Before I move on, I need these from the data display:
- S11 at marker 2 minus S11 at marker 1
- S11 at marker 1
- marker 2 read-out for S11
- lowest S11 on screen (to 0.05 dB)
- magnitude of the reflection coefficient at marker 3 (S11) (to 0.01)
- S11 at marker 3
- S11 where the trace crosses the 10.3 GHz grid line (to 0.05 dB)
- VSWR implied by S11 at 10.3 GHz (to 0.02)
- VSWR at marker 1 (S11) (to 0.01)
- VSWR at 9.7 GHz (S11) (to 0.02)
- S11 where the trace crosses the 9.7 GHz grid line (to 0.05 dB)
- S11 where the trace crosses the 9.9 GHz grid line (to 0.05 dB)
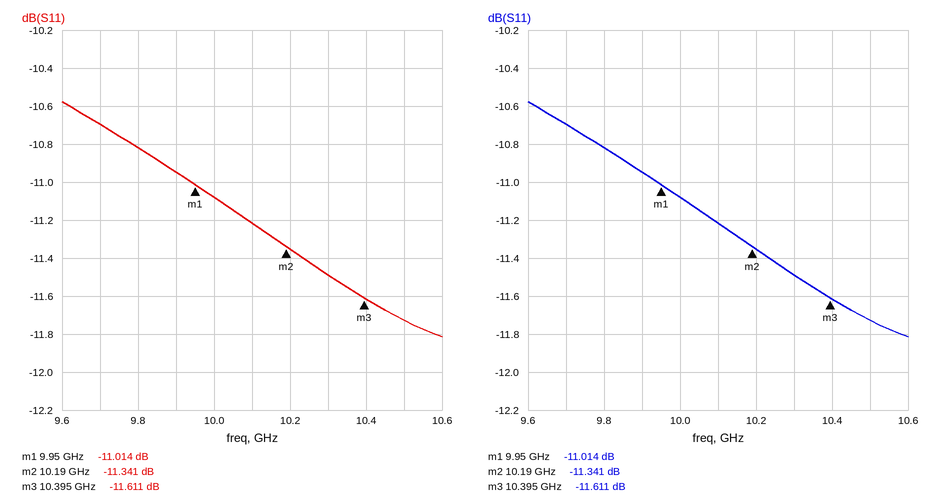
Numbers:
-0.327 dB
-11.014 dB
-11.341 dB
-11.80 dB
0.26
-11.611 dB
-11.50 dB
1.72
1.78
1.82
-10.70 dB
-10.95 dB
